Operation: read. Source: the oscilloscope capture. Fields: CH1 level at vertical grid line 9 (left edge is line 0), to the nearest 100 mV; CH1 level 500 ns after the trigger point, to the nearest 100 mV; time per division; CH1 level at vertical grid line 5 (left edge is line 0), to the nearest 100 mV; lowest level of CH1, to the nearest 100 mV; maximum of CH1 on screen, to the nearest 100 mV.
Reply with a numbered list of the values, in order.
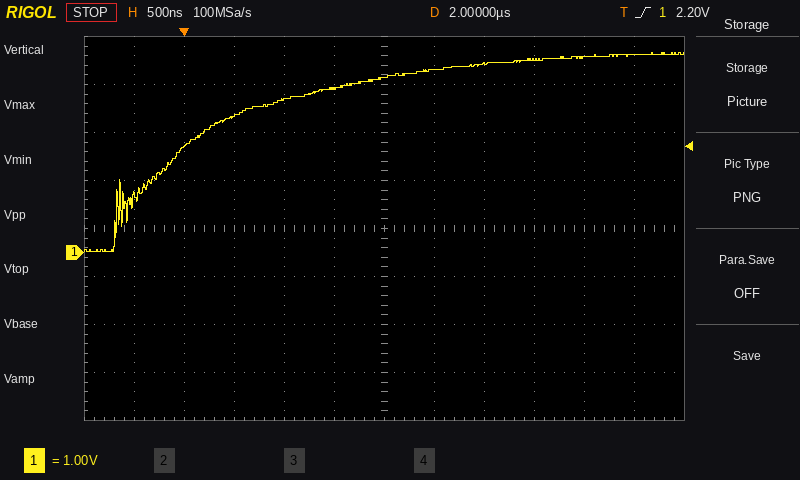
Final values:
1. 4.0 V
2. 2.8 V
3. 500 ns
4. 3.4 V
5. 0.0 V
6. 4.2 V
